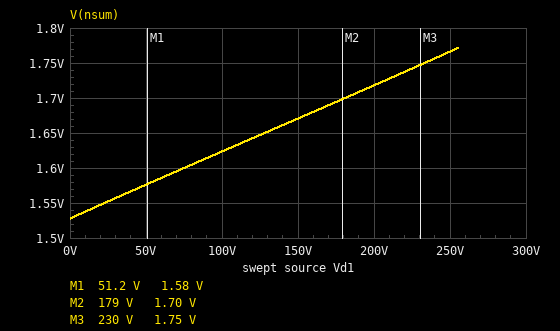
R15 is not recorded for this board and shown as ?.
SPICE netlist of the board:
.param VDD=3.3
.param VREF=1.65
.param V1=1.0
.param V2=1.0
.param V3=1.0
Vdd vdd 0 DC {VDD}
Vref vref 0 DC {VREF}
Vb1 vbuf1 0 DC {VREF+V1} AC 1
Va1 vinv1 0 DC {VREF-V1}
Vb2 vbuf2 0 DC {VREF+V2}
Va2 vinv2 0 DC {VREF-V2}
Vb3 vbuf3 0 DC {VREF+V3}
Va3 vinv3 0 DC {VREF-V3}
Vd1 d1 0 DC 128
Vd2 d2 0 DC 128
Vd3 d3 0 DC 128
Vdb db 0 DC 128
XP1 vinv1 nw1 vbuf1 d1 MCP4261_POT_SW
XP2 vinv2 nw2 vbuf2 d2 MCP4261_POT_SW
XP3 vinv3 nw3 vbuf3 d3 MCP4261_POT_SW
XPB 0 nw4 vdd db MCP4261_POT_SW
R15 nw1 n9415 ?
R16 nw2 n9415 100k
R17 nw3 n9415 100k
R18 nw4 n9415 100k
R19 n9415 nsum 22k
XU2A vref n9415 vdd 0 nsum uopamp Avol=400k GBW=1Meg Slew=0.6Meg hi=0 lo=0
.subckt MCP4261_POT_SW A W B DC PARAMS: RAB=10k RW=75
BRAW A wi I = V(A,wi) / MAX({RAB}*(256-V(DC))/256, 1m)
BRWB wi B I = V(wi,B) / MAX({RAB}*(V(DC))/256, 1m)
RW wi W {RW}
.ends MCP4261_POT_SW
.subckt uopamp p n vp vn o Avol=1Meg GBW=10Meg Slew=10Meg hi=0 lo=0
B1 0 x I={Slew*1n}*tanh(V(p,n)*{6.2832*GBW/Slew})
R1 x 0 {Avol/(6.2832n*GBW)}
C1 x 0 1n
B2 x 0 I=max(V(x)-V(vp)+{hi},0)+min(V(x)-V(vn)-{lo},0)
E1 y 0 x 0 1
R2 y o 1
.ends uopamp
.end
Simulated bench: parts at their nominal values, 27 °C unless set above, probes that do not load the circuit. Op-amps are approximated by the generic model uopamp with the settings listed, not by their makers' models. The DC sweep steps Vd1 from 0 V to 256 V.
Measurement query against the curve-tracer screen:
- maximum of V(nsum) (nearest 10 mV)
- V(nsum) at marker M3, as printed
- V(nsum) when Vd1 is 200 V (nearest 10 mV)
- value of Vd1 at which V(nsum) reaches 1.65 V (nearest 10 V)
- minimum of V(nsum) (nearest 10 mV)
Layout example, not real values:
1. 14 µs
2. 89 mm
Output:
1. 1.77 V
2. 1.75 V
3. 1.72 V
4. 130 V
5. 1.53 V
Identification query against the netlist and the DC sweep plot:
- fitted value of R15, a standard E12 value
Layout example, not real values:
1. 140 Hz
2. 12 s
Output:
1. 180 kΩ
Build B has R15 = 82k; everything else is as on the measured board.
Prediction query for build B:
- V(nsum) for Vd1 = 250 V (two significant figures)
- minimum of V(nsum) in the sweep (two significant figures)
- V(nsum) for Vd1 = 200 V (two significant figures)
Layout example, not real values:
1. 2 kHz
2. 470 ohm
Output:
1. 1.9 V
2. 1.4 V
3. 1.8 V
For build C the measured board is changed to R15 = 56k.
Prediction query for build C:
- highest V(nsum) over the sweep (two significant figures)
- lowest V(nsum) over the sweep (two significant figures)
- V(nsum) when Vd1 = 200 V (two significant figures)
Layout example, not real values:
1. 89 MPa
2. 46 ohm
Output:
1. 2.0 V
2. 1.3 V
3. 1.9 V
